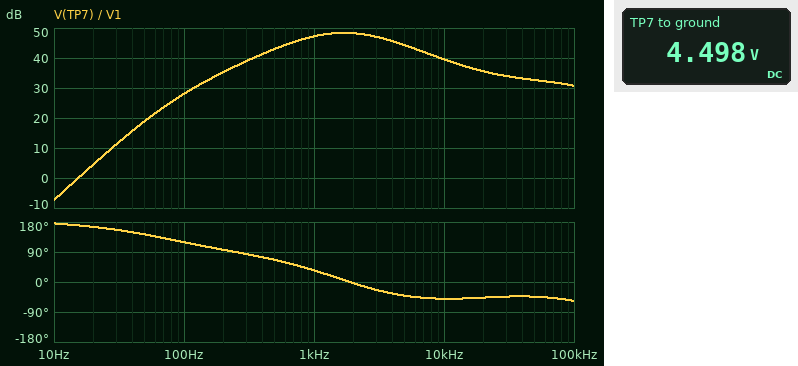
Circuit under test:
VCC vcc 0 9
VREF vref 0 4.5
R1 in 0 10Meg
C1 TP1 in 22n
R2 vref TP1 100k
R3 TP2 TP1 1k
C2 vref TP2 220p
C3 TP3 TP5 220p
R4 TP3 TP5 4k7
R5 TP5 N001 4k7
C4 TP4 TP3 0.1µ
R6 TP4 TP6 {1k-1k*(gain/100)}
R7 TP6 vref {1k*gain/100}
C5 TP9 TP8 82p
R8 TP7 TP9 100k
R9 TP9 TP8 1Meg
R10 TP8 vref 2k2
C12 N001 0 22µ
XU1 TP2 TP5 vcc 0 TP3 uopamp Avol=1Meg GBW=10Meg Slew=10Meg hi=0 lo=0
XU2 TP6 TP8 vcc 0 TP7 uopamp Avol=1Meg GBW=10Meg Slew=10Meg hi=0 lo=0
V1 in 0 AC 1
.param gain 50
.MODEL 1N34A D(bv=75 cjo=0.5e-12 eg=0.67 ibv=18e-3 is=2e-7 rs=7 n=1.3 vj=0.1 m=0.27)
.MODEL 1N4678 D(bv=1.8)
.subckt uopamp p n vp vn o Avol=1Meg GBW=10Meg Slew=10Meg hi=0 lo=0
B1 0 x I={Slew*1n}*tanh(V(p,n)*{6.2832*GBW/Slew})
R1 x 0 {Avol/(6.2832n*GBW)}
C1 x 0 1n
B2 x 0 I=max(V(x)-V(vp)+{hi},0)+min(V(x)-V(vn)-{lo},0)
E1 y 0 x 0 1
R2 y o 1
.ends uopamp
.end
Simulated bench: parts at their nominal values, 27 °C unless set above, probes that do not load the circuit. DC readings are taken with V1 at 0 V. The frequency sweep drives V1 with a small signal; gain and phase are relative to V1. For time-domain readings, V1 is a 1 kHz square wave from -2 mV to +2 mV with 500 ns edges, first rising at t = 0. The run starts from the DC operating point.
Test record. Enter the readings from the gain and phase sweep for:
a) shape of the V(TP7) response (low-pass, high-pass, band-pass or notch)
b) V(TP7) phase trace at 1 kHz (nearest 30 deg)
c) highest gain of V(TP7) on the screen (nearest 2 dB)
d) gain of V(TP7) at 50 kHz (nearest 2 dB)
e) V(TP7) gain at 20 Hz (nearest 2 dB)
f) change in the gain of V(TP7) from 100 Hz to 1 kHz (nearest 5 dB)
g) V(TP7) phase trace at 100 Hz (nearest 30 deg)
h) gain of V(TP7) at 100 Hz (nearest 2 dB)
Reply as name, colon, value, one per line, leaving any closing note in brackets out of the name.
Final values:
shape of the V(TP7) response: band-pass
V(TP7) phase trace at 1 kHz: 30 deg
highest gain of V(TP7) on the screen: 48 dB
gain of V(TP7) at 50 kHz: 32 dB
V(TP7) gain at 20 Hz: 4 dB
change in the gain of V(TP7) from 100 Hz to 1 kHz: 20 dB
V(TP7) phase trace at 100 Hz: 120 deg
gain of V(TP7) at 100 Hz: 28 dB
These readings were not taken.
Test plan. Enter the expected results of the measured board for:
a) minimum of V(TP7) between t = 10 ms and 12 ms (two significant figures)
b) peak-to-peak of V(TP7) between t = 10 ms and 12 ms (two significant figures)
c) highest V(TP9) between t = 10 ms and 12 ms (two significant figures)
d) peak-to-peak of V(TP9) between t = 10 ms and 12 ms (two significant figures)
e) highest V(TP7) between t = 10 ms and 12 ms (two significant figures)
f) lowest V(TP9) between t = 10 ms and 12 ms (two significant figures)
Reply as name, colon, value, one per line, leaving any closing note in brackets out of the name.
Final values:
minimum of V(TP7) between t = 10 ms and 12 ms: 3.7 V
peak-to-peak of V(TP7) between t = 10 ms and 12 ms: 1.5 V
highest V(TP9) between t = 10 ms and 12 ms: 5.2 V
peak-to-peak of V(TP9) between t = 10 ms and 12 ms: 1.4 V
highest V(TP7) between t = 10 ms and 12 ms: 5.3 V
lowest V(TP9) between t = 10 ms and 12 ms: 3.8 V
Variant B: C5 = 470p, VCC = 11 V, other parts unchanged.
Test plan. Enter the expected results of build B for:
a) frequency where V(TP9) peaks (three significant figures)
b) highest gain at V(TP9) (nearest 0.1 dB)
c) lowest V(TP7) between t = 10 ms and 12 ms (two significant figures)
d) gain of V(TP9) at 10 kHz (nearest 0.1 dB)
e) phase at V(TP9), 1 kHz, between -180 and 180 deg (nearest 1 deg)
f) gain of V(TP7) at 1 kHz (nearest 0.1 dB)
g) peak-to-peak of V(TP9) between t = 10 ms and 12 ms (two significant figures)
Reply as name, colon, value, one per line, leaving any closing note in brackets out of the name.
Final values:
frequency where V(TP9) peaks: 741 Hz
highest gain at V(TP9): 37.8 dB
lowest V(TP7) between t = 10 ms and 12 ms: 4.3 V
gain of V(TP9) at 10 kHz: 23.4 dB
phase at V(TP9), 1 kHz, between -180 and 180 deg: -10 deg
gain of V(TP7) at 1 kHz: 38.7 dB
peak-to-peak of V(TP9) between t = 10 ms and 12 ms: 350 mV
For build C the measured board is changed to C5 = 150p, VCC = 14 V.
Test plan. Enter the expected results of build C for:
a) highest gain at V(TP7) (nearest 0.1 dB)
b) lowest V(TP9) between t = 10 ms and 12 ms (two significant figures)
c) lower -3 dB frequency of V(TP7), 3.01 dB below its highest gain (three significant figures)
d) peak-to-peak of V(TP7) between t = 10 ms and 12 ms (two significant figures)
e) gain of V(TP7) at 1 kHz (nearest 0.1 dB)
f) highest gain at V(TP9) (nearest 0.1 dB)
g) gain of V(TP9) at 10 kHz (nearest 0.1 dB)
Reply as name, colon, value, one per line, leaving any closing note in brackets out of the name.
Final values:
highest gain at V(TP7): 45.7 dB
lowest V(TP9) between t = 10 ms and 12 ms: 4.0 V
lower -3 dB frequency of V(TP7), 3.01 dB below its highest gain: 526 Hz
peak-to-peak of V(TP7) between t = 10 ms and 12 ms: 1.1 V
gain of V(TP7) at 1 kHz: 45.5 dB
highest gain at V(TP9): 44.9 dB
gain of V(TP9) at 10 kHz: 33.0 dB
